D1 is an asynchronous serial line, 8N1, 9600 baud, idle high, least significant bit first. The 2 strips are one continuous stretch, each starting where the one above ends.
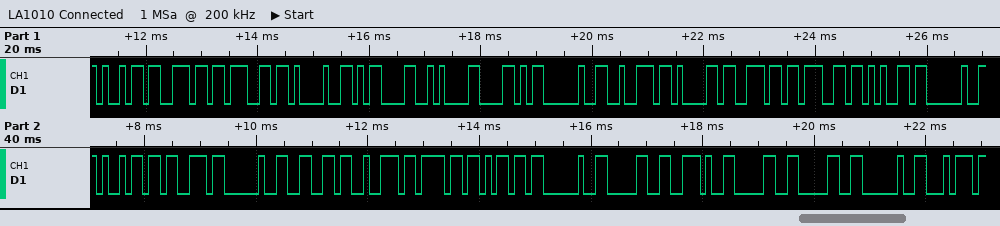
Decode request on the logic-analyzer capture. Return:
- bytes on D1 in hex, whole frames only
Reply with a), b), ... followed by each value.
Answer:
a) 0x69 0x6E 0x67 0x21 0x0D 0x0A 0x58 0x20 0x72 0x61 0x6E 0x67 0x65 0x20 0x69 0x73 0x20 0x66 0x72 0x6F 0x6D 0x20 0x30 0x2E 0x30 0x30 0x20 0x74
